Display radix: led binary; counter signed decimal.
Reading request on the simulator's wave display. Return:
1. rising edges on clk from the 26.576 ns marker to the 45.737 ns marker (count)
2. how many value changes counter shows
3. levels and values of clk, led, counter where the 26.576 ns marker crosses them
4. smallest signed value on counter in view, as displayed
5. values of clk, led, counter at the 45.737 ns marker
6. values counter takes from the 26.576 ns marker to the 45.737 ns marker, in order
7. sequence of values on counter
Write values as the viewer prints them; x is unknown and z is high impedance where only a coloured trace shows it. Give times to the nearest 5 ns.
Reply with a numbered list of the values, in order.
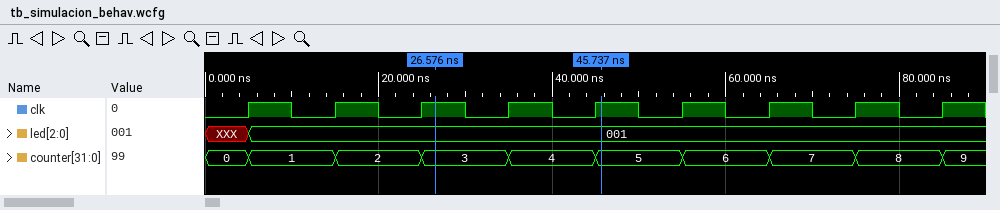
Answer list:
1. 2
2. 9
3. clk=1, led=001, counter=3
4. 0
5. clk=1, led=001, counter=5
6. 3, 4, 5
7. 0, 1, 2, 3, 4, 5, 6, 7, 8, 9
